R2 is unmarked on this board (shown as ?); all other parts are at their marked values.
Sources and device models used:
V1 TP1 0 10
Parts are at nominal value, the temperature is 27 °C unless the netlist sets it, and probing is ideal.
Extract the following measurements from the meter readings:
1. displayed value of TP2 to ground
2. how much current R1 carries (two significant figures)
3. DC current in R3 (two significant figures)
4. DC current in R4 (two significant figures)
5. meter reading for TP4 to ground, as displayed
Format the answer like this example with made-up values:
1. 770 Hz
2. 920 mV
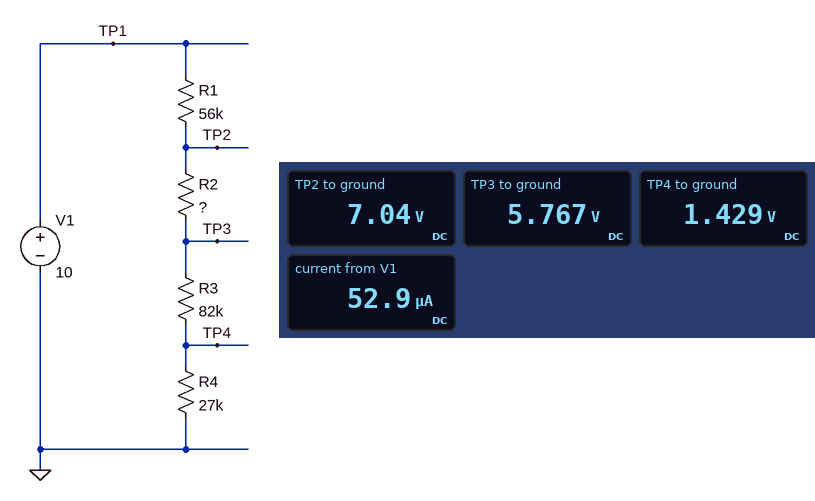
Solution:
1. 7.04 V
2. 53 µA
3. 53 µA
4. 53 µA
5. 1.429 V
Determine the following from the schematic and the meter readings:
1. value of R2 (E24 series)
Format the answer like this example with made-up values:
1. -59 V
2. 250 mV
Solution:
1. 24 kΩ
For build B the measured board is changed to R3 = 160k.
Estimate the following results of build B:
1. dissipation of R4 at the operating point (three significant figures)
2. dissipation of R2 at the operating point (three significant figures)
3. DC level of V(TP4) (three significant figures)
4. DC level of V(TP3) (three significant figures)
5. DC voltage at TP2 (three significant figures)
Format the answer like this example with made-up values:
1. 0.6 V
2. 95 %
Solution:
1. 37.9 µW
2. 33.7 µW
3. 1.01 V
4. 7.00 V
5. 7.90 V
